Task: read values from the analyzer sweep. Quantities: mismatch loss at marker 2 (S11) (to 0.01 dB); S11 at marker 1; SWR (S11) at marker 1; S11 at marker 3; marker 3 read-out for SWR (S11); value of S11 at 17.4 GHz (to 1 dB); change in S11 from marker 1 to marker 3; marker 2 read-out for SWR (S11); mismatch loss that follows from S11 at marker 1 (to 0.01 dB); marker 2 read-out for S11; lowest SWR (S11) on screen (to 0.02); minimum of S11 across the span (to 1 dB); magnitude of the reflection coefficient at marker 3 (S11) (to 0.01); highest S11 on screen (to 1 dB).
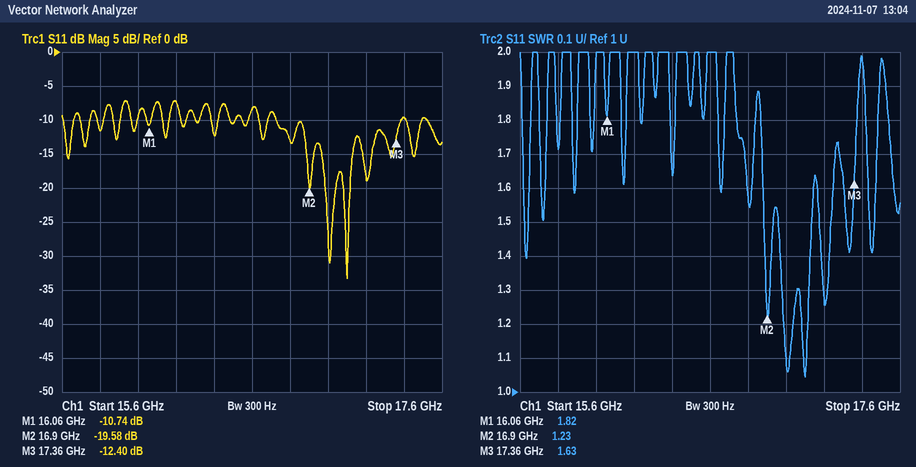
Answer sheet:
0.05 dB
-10.74 dB
1.82
-12.40 dB
1.63
-10 dB
-1.66 dB
1.23
0.38 dB
-19.58 dB
1.04
-33 dB
0.24
-7 dB
